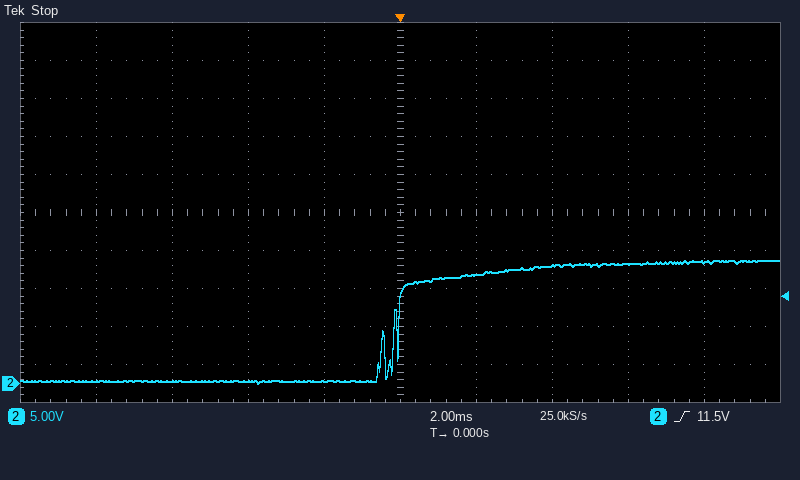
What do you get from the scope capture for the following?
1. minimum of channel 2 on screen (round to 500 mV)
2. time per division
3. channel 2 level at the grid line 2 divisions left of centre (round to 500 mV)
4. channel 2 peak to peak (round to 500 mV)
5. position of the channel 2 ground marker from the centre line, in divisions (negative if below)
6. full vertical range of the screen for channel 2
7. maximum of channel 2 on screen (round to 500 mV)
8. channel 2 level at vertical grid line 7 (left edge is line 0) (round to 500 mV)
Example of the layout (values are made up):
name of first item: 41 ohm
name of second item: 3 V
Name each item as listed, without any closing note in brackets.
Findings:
minimum of channel 2 on screen: 0.0 V
time per division: 2 ms
channel 2 level at the grid line 2 divisions left of centre: 500 mV
channel 2 peak to peak: 16.0 V
position of the channel 2 ground marker from the centre line, in divisions: -4.5 div
full vertical range of the screen for channel 2: 50 V
maximum of channel 2 on screen: 16.0 V
channel 2 level at vertical grid line 7 (left edge is line 0): 15.5 V
